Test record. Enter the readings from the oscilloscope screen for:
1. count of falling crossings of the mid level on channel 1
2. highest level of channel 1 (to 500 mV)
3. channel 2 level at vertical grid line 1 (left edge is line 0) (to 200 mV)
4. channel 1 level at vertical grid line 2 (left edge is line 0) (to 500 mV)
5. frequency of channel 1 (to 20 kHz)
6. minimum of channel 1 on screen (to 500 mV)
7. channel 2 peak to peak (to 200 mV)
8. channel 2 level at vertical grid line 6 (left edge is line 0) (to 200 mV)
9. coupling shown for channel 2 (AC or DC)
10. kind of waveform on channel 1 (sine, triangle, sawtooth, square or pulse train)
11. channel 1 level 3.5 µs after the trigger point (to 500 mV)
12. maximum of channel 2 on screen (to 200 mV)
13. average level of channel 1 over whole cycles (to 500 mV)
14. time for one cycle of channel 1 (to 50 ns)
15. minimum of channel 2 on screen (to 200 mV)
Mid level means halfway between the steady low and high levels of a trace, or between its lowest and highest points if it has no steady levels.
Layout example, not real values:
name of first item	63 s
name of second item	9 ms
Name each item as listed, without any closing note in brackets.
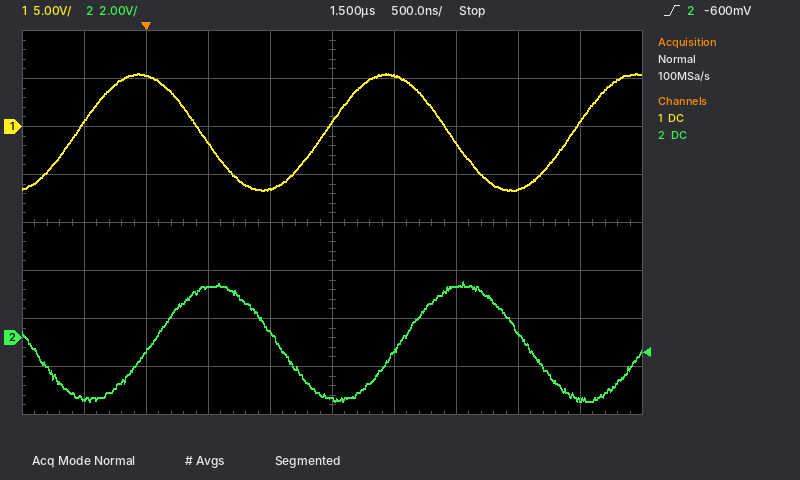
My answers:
count of falling crossings of the mid level on channel 1	2
highest level of channel 1	5.5 V
channel 2 level at vertical grid line 1 (left edge is line 0)	-2.6 V
channel 1 level at vertical grid line 2 (left edge is line 0)	5.5 V
frequency of channel 1	500 kHz
minimum of channel 1 on screen	-6.5 V
channel 2 peak to peak	5.0 V
channel 2 level at vertical grid line 6 (left edge is line 0)	-600 mV
coupling shown for channel 2	DC
kind of waveform on channel 1	sine
channel 1 level 3.5 µs after the trigger point	500 mV
maximum of channel 2 on screen	2.4 V
average level of channel 1 over whole cycles	-500 mV
time for one cycle of channel 1	2.00 µs
minimum of channel 2 on screen	-2.6 V
